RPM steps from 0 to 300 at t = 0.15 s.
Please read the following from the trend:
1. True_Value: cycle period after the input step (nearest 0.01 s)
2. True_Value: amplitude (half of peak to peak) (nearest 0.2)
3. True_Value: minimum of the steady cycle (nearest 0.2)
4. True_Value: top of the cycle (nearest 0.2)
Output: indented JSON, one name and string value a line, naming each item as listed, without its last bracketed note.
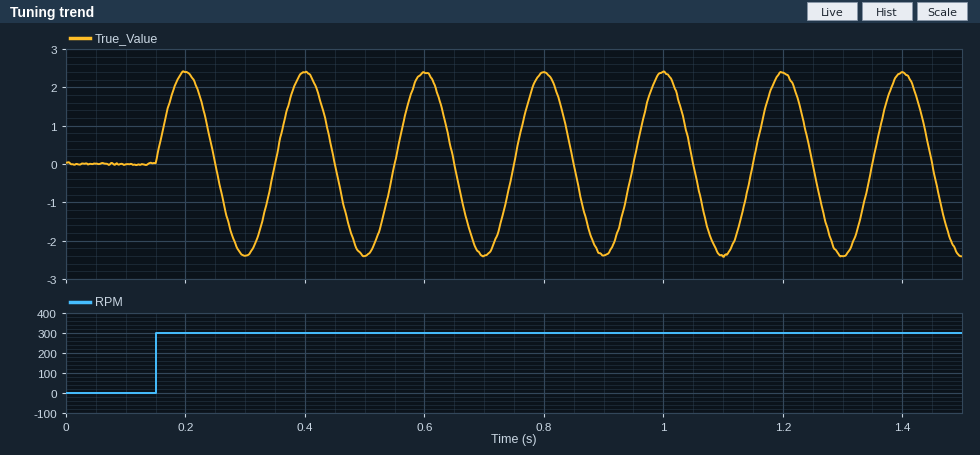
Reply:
{
  "True_Value: cycle period after the input step": "0.20 s",
  "True_Value: amplitude (half of peak to peak)": "2.4",
  "True_Value: minimum of the steady cycle": "-2.4",
  "True_Value: top of the cycle": "2.4"
}
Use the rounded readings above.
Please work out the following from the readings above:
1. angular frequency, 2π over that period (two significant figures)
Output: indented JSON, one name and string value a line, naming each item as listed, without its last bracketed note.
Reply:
{
  "angular frequency, 2π over that period": "31 rad/s"
}
